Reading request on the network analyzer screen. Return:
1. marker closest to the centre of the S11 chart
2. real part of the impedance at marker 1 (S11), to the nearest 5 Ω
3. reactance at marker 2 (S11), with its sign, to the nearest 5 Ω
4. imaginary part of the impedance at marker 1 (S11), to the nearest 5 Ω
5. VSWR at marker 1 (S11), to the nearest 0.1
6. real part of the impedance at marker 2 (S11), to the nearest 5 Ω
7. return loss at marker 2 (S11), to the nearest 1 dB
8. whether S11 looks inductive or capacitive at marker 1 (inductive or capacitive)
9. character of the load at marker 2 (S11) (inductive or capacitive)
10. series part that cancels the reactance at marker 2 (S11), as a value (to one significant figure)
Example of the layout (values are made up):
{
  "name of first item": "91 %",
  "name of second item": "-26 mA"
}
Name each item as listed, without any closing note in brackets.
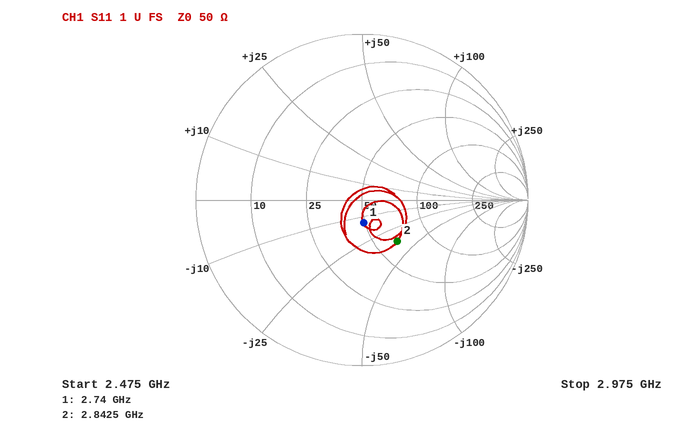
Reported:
{
  "marker closest to the centre of the S11 chart": "marker 1",
  "real part of the impedance at marker 1 (S11), to the nearest 5 Ω": "50 Ω",
  "reactance at marker 2 (S11), with its sign, to the nearest 5 Ω": "-35 Ω",
  "imaginary part of the impedance at marker 1 (S11), to the nearest 5 Ω": "-15 Ω",
  "VSWR at marker 1 (S11), to the nearest 0.1": "1.3",
  "real part of the impedance at marker 2 (S11), to the nearest 5 Ω": "65 Ω",
  "return loss at marker 2 (S11), to the nearest 1 dB": "10 dB",
  "whether S11 looks inductive or capacitive at marker 1": "capacitive",
  "character of the load at marker 2 (S11)": "capacitive",
  "series part that cancels the reactance at marker 2 (S11), as a value": "2 nH"
}
